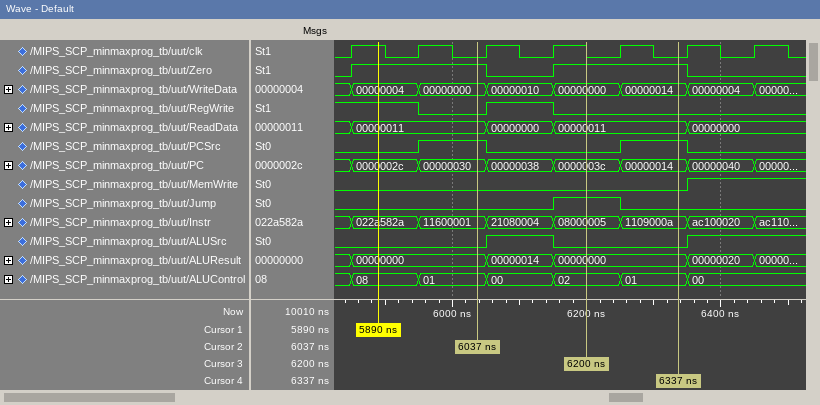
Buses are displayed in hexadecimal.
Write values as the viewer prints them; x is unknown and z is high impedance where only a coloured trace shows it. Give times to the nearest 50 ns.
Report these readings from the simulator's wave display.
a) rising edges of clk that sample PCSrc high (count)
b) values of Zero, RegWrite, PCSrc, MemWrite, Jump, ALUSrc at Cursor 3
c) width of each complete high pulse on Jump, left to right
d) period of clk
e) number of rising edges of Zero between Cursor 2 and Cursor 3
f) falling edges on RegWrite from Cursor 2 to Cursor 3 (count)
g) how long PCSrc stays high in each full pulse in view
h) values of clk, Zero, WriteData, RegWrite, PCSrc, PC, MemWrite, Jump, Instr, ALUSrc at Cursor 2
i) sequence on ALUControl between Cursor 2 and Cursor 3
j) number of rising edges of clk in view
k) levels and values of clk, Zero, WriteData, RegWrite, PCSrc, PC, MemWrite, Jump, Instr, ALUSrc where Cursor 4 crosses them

2
Zero=1, RegWrite=0, PCSrc=0, MemWrite=0, Jump=1, ALUSrc=0
100 ns
100 ns
1
1
100 ns, 100 ns
clk=0, Zero=1, WriteData=00000000, RegWrite=0, PCSrc=1, PC=00000030, MemWrite=0, Jump=0, Instr=11600001, ALUSrc=0
01, 00, 02
7
clk=0, Zero=1, WriteData=00000014, RegWrite=0, PCSrc=1, PC=00000014, MemWrite=0, Jump=0, Instr=1109000a, ALUSrc=0
